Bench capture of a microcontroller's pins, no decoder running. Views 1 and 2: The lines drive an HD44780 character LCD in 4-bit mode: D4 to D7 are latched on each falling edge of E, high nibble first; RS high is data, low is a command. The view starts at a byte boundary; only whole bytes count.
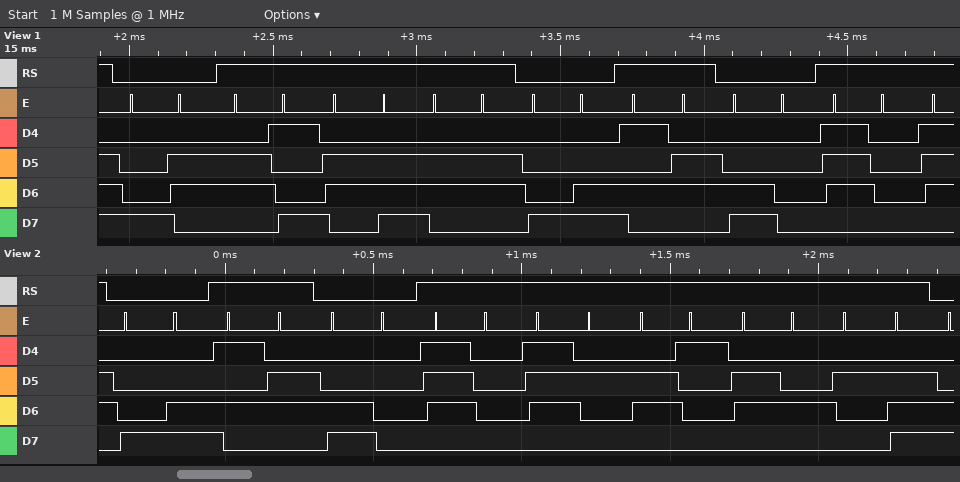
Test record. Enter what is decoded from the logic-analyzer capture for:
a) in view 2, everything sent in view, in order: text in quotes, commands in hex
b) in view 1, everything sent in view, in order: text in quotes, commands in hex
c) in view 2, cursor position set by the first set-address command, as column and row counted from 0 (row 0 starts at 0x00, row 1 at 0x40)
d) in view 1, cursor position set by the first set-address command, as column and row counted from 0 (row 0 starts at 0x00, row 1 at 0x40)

0x8C "V" 0xC0 "prad."
0x86 "inf" 0x8C "V" 0xC0 "p"
column 12, row 0
column 6, row 0
